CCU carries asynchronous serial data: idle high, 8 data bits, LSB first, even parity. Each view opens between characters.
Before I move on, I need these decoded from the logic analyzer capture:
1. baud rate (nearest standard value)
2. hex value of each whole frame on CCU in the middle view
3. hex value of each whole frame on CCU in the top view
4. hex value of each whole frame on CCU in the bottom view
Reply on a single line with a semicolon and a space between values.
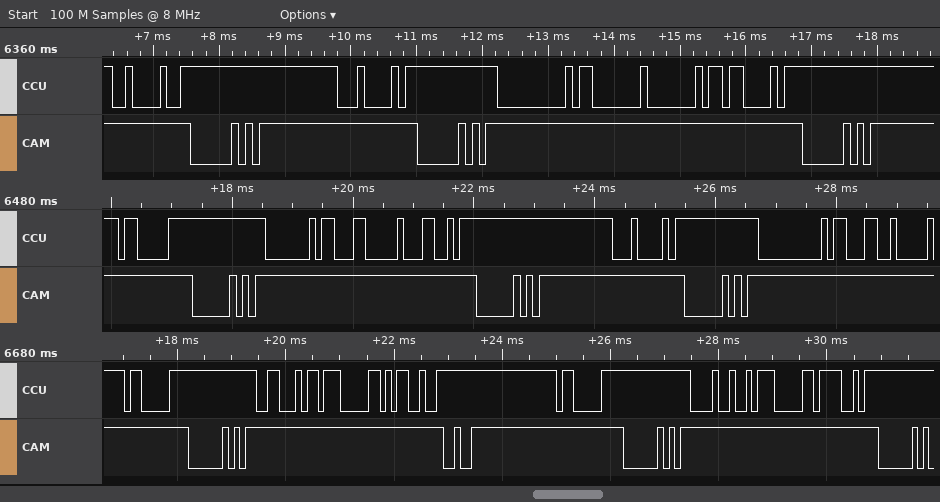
9600 baud; 83, 40, 0C, 4C, 84, 00, 63; 42, 84, 00, 03, 40, 43; 83, 46, 07, 4D, 83, 48, 07, 4F
